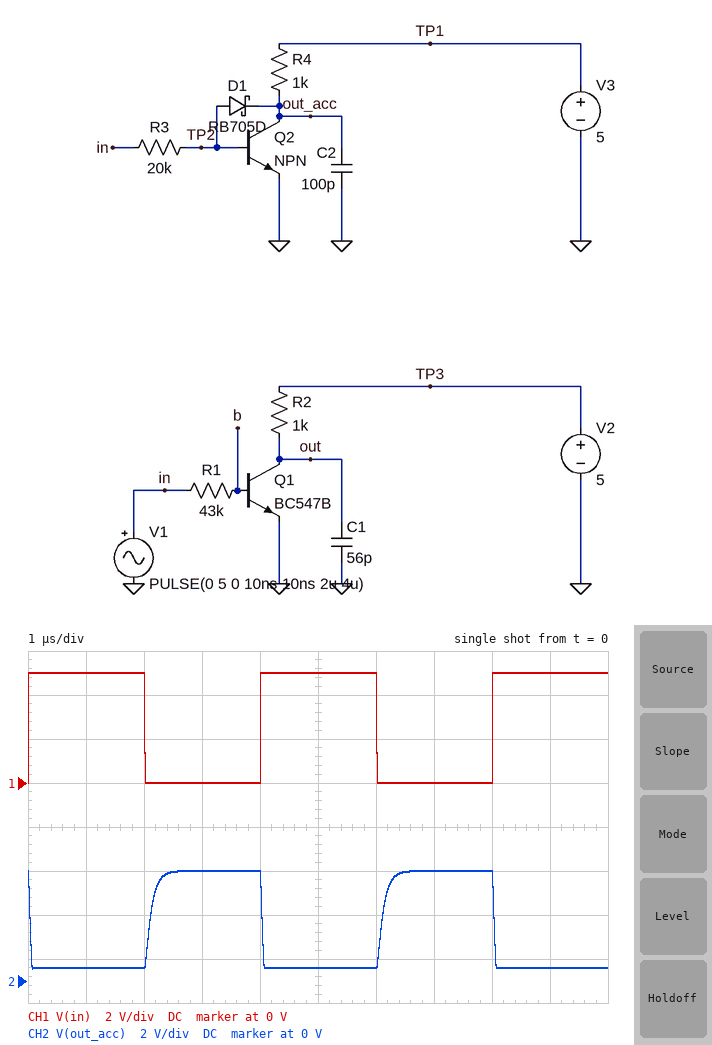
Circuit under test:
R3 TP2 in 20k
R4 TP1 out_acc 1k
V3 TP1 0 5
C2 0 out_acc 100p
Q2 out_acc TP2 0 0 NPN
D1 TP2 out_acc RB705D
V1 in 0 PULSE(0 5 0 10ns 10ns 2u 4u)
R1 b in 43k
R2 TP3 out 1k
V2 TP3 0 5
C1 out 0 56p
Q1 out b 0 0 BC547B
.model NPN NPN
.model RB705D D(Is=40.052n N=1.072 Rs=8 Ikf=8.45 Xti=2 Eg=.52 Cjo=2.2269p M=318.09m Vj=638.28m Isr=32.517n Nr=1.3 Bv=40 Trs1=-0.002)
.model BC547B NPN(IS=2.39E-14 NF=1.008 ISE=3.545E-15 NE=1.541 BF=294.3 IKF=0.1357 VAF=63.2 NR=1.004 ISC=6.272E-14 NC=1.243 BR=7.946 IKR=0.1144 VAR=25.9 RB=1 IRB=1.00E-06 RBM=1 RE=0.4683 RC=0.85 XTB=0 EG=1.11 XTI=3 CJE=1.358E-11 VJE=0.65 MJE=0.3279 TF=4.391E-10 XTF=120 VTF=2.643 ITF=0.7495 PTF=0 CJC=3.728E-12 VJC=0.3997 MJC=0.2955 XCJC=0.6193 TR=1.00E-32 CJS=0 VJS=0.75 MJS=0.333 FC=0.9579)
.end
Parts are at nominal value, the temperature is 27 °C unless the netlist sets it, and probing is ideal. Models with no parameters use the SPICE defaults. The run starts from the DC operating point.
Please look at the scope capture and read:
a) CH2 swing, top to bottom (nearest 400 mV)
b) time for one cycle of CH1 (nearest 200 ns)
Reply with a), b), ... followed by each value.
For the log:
a) 4.4 V
b) 4.0 µs
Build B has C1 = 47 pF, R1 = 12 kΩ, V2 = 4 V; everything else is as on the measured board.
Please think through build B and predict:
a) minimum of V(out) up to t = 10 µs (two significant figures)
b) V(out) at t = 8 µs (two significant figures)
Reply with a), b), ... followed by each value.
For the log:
a) 37 mV
b) 4.0 V
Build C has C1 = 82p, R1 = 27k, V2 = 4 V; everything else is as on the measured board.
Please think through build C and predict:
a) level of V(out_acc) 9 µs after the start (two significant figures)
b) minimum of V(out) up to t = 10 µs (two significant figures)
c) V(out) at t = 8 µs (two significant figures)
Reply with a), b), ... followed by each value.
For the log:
a) 590 mV
b) 53 mV
c) 4.0 V
